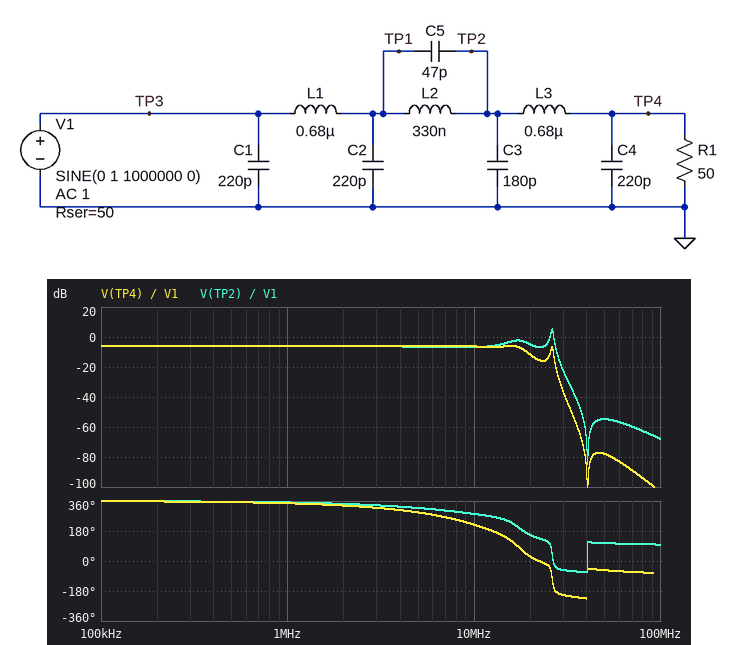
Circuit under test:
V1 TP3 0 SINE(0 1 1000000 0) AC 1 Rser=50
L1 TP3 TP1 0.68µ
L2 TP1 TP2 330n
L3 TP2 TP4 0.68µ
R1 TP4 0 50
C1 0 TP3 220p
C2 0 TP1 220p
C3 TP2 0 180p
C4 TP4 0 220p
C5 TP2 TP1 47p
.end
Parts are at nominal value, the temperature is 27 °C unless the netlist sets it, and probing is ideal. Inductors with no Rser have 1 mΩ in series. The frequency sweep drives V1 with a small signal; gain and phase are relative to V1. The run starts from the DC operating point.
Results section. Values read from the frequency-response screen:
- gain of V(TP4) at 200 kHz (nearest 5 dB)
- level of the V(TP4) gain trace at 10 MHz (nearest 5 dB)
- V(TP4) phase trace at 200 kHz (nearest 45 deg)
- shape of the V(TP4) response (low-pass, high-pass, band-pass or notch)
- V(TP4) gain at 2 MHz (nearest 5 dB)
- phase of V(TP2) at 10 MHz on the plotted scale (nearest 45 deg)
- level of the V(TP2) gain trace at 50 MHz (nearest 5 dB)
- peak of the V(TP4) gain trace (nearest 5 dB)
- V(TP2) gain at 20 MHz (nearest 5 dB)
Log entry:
-5 dB
-5 dB
360 deg
low-pass
-5 dB
270 deg
-55 dB
-5 dB
-5 dB
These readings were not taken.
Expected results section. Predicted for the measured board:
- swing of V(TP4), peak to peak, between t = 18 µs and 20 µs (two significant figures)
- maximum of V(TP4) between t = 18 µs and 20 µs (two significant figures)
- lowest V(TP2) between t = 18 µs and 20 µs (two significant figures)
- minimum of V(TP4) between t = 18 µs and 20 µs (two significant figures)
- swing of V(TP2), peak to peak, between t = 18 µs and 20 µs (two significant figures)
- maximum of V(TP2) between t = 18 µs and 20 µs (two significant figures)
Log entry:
1.0 V
500 mV
-500 mV
-500 mV
1.0 V
500 mV
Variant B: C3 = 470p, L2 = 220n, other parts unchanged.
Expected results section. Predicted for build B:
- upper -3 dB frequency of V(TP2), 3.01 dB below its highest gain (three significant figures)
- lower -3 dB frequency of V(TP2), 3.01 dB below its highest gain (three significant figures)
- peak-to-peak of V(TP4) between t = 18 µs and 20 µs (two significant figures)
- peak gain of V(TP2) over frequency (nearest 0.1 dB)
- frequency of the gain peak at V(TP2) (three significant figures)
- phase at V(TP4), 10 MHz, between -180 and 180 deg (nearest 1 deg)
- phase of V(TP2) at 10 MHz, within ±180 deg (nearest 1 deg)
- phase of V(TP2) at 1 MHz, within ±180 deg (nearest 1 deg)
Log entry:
27.1 MHz
26.5 MHz
1.0 V
2.5 dB
26.8 MHz
-161 deg
-97 deg
-11 deg
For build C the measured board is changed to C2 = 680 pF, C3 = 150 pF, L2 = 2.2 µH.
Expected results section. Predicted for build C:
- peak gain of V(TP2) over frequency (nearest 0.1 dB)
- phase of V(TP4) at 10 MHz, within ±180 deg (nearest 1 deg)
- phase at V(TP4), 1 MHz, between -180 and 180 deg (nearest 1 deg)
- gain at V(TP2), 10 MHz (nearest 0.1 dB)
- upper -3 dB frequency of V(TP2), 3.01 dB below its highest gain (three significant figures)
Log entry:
-6.0 dB
112 deg
-24 deg
-19.1 dB
5.32 MHz
